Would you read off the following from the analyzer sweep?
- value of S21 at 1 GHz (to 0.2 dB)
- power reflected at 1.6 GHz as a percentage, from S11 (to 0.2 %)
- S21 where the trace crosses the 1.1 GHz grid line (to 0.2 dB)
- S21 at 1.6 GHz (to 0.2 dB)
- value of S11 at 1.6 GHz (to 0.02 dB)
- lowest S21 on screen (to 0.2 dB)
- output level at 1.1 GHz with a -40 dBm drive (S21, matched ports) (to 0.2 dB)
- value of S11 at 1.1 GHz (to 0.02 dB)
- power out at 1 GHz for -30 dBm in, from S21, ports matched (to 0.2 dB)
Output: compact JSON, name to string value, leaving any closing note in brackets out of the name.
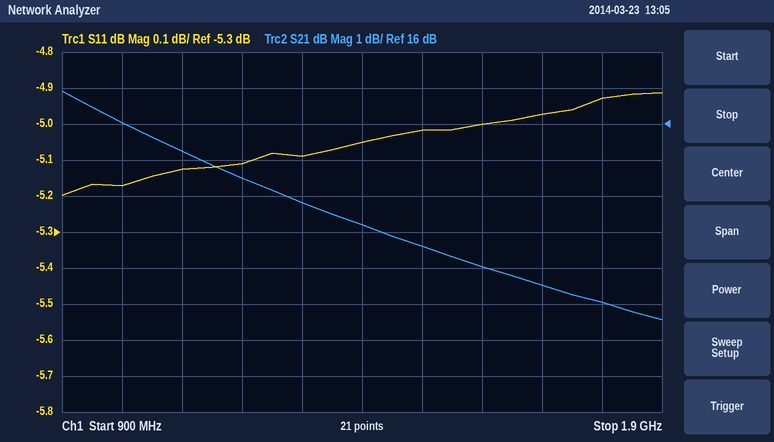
{"value of S21 at 1 GHz": "16.0 dB", "power reflected at 1.6 GHz as a percentage, from S11": "31.6 %", "S21 where the trace crosses the 1.1 GHz grid line": "15.2 dB", "S21 at 1.6 GHz": "12.0 dB", "value of S11 at 1.6 GHz": "-5.00 dB", "lowest S21 on screen": "10.6 dB", "output level at 1.1 GHz with a -40 dBm drive (S21, matched ports)": "-24.8 dBm", "value of S11 at 1.1 GHz": "-5.12 dB", "power out at 1 GHz for -30 dBm in, from S21, ports matched": "-14.0 dBm"}
